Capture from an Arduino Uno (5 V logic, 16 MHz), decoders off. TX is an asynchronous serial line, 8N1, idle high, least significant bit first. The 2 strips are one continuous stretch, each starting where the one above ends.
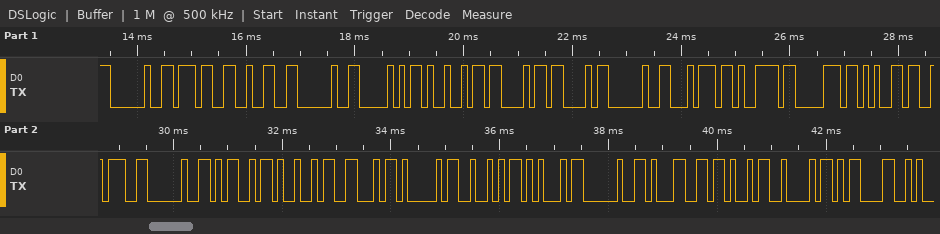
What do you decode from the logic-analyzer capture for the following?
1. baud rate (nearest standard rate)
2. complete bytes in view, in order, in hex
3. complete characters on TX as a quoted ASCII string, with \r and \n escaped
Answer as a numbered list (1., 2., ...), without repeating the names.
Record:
1. 9600 baud
2. 20 37 32 20 50 49 43 43 20 74 79 70 65 3A 20 4D 49 46 41 52 45 20 31 4B 42 0D
3. " 72 PICC type: MIFARE 1KB\r"
